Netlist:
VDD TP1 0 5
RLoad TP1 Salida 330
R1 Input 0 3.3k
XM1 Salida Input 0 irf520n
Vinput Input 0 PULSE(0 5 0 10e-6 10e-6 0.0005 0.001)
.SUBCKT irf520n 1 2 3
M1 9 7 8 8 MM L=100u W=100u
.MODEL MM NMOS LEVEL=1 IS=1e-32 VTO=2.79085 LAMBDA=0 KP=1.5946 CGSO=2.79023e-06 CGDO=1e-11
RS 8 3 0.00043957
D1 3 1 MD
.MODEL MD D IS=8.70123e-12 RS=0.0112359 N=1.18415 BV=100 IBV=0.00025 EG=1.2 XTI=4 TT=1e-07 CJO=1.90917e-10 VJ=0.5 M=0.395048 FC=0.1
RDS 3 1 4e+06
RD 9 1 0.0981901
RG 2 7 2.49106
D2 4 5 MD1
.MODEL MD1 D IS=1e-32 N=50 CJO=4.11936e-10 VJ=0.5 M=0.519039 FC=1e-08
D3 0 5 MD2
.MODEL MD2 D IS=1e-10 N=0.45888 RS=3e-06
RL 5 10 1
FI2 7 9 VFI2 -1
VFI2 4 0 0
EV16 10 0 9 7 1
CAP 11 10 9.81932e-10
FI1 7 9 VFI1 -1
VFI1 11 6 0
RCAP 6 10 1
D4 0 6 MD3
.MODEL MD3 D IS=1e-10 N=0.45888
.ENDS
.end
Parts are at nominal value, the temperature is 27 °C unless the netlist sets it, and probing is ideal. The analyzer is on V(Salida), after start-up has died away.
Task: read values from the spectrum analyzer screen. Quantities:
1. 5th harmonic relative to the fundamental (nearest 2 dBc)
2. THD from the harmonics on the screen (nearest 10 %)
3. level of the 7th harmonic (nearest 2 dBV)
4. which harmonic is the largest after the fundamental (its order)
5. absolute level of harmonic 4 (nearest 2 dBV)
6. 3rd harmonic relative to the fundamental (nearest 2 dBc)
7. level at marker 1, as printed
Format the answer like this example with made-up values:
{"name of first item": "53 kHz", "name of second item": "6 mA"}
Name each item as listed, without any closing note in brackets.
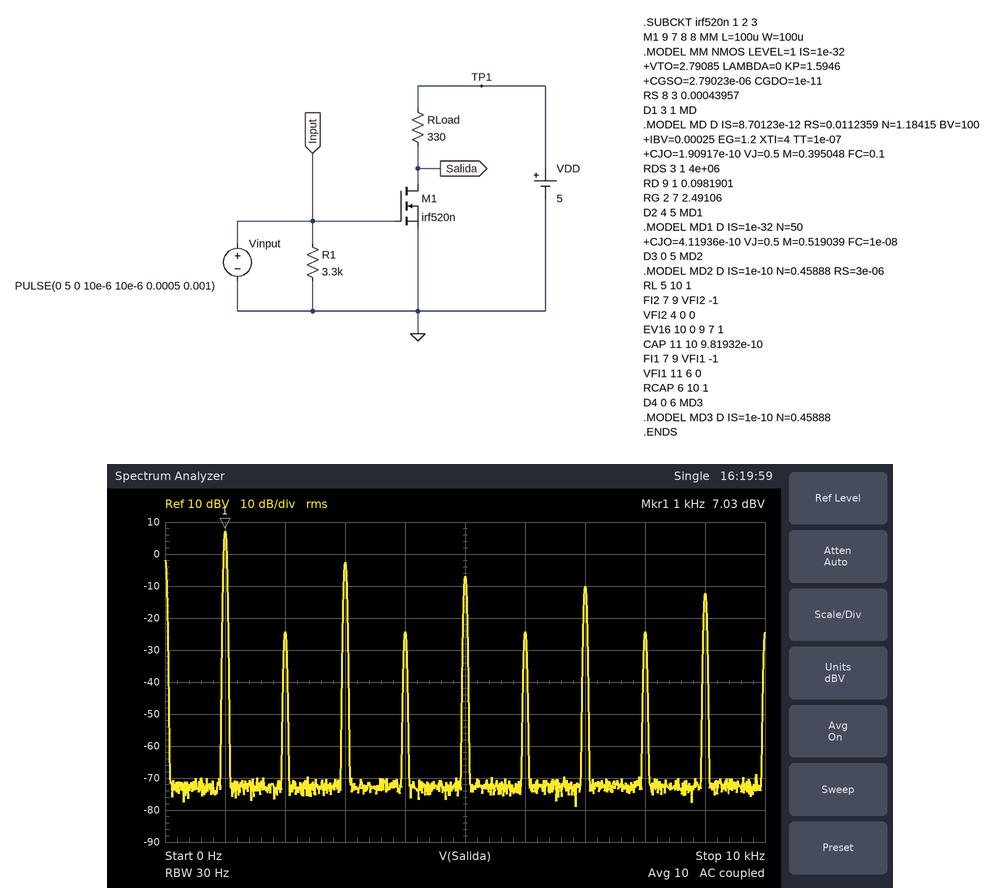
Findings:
{"5th harmonic relative to the fundamental": "-14 dBc", "THD from the harmonics on the screen": "40 %", "level of the 7th harmonic": "-10 dBV", "which harmonic is the largest after the fundamental": "3", "absolute level of harmonic 4": "-24 dBV", "3rd harmonic relative to the fundamental": "-10 dBc", "level at marker 1, as printed": "7.03 dBV"}
